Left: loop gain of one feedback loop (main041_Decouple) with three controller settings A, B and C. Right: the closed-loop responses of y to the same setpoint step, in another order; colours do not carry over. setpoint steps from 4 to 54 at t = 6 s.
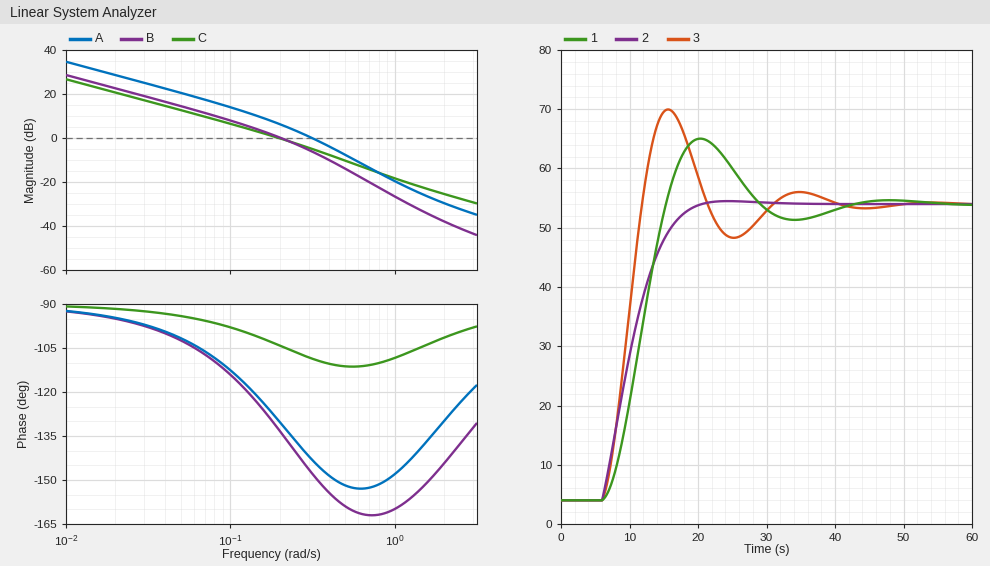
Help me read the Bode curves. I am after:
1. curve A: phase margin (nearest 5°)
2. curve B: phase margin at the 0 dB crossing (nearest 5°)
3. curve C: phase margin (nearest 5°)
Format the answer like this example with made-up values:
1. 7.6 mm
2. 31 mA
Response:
1. 35°
2. 45°
3. 75°
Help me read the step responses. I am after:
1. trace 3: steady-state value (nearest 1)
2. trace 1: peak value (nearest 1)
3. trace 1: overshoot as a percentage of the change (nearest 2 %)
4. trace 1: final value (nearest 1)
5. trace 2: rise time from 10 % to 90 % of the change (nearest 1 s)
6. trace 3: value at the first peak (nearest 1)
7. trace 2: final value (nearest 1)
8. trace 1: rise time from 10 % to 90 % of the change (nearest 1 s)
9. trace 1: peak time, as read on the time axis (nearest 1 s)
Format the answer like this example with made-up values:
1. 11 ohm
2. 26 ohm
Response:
1. 54
2. 65
3. 22 %
4. 54
5. 9 s
6. 70
7. 54
8. 6 s
9. 20 s
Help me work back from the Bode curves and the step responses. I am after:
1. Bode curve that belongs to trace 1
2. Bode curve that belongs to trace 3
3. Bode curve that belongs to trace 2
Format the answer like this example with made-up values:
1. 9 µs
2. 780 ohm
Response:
1. B
2. A
3. C
